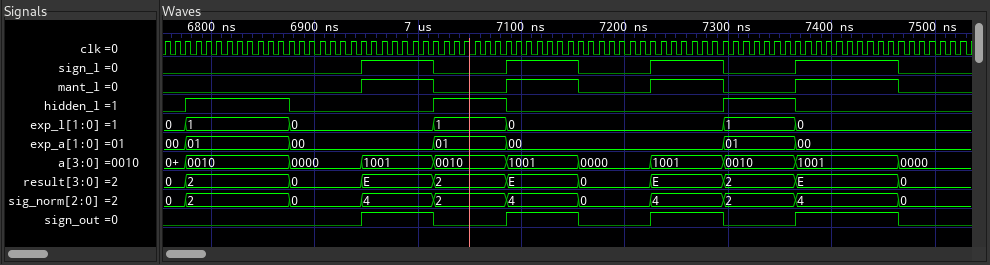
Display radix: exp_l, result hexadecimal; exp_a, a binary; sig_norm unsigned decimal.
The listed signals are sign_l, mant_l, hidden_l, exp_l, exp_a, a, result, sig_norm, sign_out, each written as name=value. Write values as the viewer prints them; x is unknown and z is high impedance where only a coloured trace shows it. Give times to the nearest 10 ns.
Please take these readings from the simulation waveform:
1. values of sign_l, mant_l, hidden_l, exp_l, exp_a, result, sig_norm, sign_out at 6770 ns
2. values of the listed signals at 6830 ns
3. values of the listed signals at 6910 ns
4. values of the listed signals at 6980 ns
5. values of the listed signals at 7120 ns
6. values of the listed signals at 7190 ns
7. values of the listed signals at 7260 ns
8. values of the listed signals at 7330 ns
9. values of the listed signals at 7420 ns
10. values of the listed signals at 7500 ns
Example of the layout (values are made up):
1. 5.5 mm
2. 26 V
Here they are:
1. sign_l=0, mant_l=0, hidden_l=0, exp_l=0, exp_a=00, result=0, sig_norm=0, sign_out=0
2. sign_l=0, mant_l=0, hidden_l=1, exp_l=1, exp_a=01, a=0010, result=2, sig_norm=2, sign_out=0
3. sign_l=0, mant_l=0, hidden_l=0, exp_l=0, exp_a=00, a=0000, result=0, sig_norm=0, sign_out=0
4. sign_l=1, mant_l=1, hidden_l=0, exp_l=0, exp_a=00, a=1001, result=E, sig_norm=4, sign_out=1
5. sign_l=1, mant_l=1, hidden_l=0, exp_l=0, exp_a=00, a=1001, result=E, sig_norm=4, sign_out=1
6. sign_l=0, mant_l=0, hidden_l=0, exp_l=0, exp_a=00, a=0000, result=0, sig_norm=0, sign_out=0
7. sign_l=1, mant_l=1, hidden_l=0, exp_l=0, exp_a=00, a=1001, result=E, sig_norm=4, sign_out=1
8. sign_l=0, mant_l=0, hidden_l=1, exp_l=1, exp_a=01, a=0010, result=2, sig_norm=2, sign_out=0
9. sign_l=1, mant_l=1, hidden_l=0, exp_l=0, exp_a=00, a=1001, result=E, sig_norm=4, sign_out=1
10. sign_l=0, mant_l=0, hidden_l=0, exp_l=0, exp_a=00, a=0000, result=0, sig_norm=0, sign_out=0
